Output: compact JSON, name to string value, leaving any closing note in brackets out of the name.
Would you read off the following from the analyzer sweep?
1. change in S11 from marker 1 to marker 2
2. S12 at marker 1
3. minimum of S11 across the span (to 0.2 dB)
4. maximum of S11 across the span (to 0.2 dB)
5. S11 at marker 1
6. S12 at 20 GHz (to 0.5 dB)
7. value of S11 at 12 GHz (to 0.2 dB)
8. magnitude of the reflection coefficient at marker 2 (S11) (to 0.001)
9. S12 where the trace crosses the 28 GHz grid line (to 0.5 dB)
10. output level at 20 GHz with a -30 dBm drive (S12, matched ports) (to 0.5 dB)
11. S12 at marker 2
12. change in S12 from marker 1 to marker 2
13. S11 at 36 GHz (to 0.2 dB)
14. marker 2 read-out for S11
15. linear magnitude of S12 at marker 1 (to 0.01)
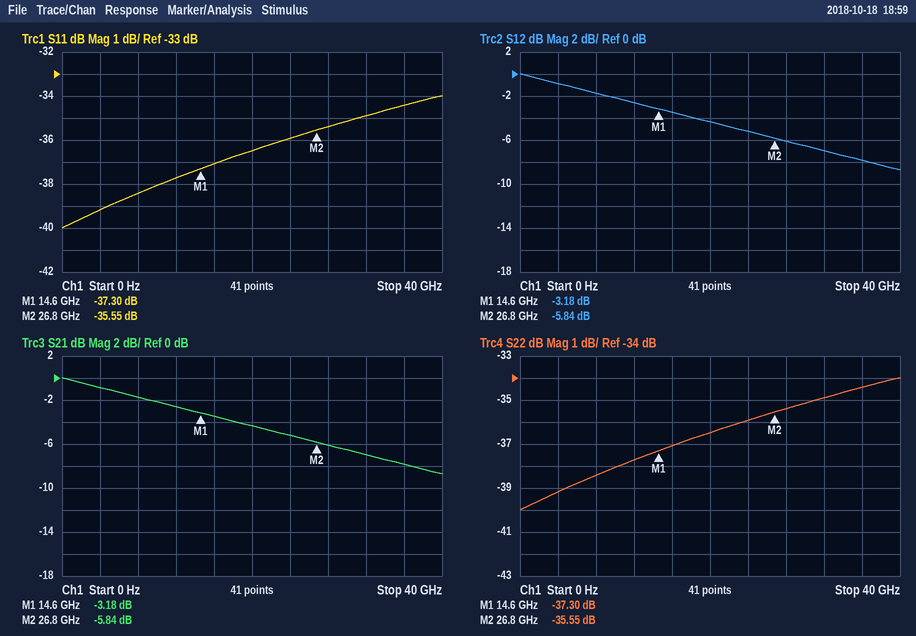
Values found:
{"change in S11 from marker 1 to marker 2": "1.75 dB", "S12 at marker 1": "-3.18 dB", "minimum of S11 across the span": "-40.0 dB", "maximum of S11 across the span": "-34.0 dB", "S11 at marker 1": "-37.30 dB", "S12 at 20 GHz": "-4.5 dB", "value of S11 at 12 GHz": "-37.8 dB", "magnitude of the reflection coefficient at marker 2 (S11)": "0.017", "S12 where the trace crosses the 28 GHz grid line": "-6.0 dB", "output level at 20 GHz with a -30 dBm drive (S12, matched ports)": "-34.5 dBm", "S12 at marker 2": "-5.84 dB", "change in S12 from marker 1 to marker 2": "-2.66 dB", "S11 at 36 GHz": "-34.4 dB", "marker 2 read-out for S11": "-35.55 dB", "linear magnitude of S12 at marker 1": "0.69"}
